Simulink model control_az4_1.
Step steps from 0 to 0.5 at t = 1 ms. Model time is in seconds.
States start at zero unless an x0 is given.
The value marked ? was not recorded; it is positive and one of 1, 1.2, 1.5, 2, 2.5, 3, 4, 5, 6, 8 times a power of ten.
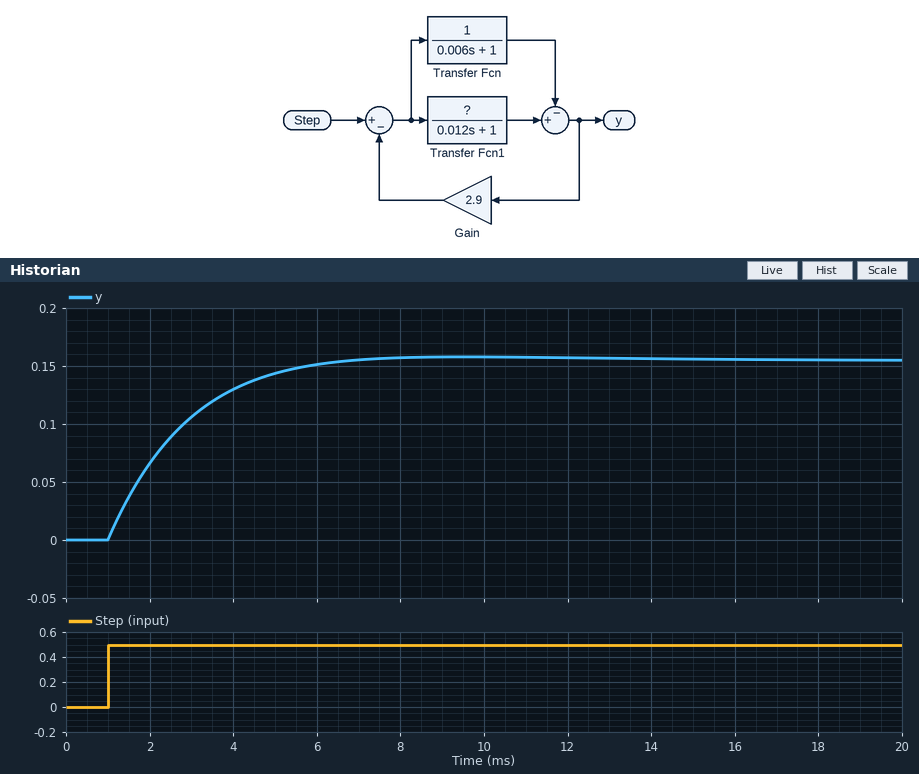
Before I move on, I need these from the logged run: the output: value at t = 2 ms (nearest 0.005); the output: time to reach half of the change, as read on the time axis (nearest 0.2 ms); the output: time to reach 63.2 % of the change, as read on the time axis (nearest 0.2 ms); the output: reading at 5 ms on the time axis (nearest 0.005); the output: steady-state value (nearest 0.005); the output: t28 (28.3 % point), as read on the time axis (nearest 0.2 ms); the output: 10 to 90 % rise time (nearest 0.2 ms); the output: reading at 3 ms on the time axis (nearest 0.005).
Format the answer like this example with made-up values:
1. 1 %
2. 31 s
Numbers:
1. 0.065
2. 2.2 ms
3. 2.8 ms
4. 0.145
5. 0.155
6. 1.6 ms
7. 3.4 ms
8. 0.105
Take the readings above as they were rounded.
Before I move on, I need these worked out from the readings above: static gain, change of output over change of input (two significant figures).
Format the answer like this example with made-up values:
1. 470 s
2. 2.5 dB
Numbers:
1. 0.31
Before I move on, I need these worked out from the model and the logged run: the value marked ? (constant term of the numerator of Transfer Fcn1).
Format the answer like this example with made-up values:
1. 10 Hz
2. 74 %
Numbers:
1. 4
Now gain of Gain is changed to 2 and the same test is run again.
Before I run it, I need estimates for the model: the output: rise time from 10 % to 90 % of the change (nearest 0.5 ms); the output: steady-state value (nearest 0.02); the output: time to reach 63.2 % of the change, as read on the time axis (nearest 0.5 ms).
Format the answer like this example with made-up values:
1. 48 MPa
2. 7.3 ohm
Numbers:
1. 4.5 ms
2. 0.22
3. 3.5 ms
